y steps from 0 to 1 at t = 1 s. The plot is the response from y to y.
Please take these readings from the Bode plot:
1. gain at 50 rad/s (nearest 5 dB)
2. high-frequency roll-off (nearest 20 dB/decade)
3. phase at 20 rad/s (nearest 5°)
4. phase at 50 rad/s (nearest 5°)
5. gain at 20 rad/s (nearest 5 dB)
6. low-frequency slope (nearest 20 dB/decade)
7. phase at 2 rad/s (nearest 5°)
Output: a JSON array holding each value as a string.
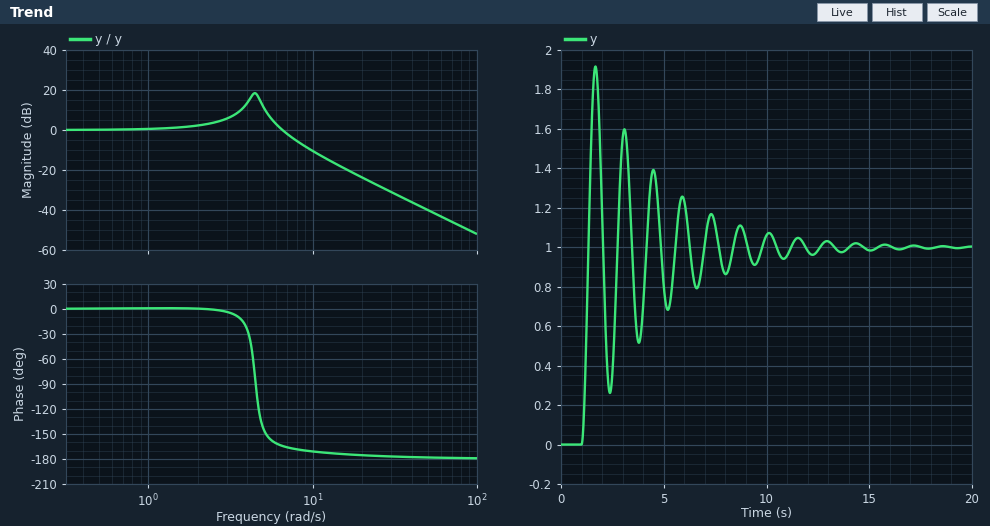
["-40 dB", "-40 dB/decade", "-175°", "-180°", "-25 dB", "0 dB/decade", "0°"]
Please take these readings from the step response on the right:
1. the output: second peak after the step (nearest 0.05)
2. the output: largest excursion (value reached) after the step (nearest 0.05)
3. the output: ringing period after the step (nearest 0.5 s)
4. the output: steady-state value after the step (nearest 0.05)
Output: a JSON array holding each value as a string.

["1.60", "1.90", "1.5 s", "1.00"]
